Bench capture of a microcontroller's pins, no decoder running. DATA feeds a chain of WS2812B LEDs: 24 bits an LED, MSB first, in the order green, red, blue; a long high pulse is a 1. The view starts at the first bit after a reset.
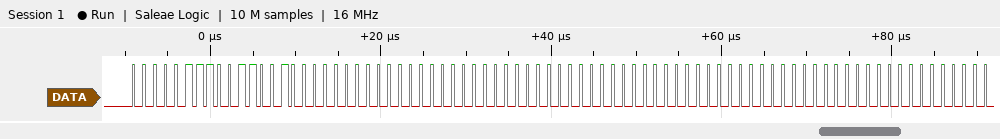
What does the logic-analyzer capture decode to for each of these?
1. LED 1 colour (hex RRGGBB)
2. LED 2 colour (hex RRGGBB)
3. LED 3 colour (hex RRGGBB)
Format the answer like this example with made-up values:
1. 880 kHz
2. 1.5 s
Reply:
1. #320700
2. #000000
3. #000000
